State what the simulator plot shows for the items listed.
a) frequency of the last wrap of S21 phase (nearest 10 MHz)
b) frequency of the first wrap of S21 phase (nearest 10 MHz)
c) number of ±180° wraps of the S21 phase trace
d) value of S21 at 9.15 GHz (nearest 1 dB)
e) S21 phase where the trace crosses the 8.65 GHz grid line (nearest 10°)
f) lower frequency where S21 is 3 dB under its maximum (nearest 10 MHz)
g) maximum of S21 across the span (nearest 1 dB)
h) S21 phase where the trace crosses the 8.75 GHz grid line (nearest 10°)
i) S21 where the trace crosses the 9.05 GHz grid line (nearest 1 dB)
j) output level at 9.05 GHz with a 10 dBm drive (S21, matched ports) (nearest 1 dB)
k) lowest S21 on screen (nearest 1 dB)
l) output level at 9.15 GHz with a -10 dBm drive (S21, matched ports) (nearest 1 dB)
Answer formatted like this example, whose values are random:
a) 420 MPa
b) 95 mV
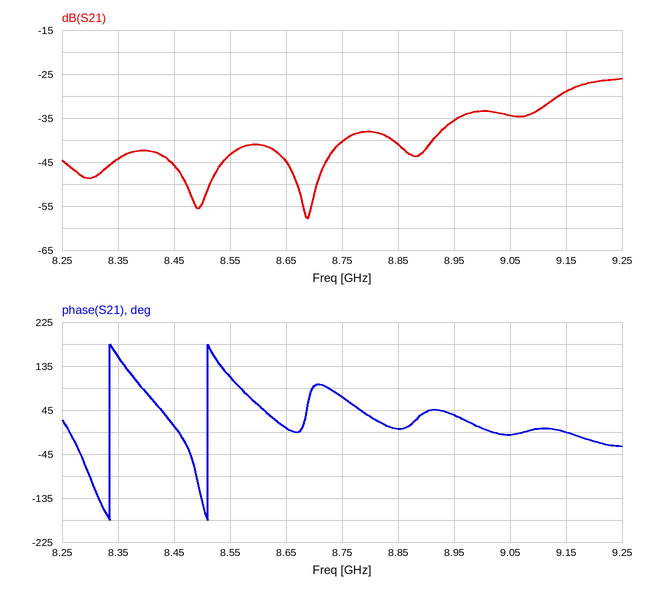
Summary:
a) 8.51 GHz
b) 8.34 GHz
c) 2
d) -29 dB
e) 10°
f) 9.15 GHz
g) -26 dB
h) 70°
i) -34 dB
j) -24 dBm
k) -58 dB
l) -39 dBm
